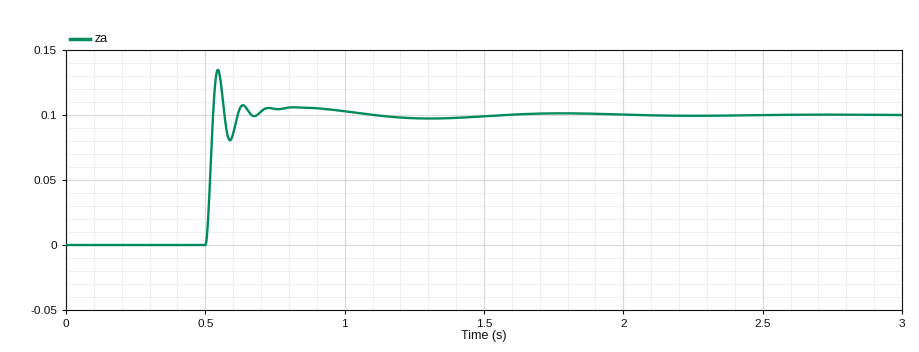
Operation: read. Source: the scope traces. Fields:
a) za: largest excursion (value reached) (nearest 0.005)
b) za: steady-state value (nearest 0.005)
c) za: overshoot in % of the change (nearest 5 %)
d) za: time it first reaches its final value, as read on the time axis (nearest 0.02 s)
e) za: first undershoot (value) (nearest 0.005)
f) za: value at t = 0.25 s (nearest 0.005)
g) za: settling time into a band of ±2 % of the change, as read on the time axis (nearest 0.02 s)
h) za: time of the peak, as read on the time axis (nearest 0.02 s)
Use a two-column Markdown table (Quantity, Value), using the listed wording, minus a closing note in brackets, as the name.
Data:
| Quantity | Value |
|---|---|
| za: largest excursion (value reached) | 0.135 |
| za: steady-state value | 0.100 |
| za: overshoot in % of the change | 35 % |
| za: time it first reaches its final value, as read on the time axis | 0.52 s |
| za: first undershoot (value) | 0.080 |
| za: value at t = 0.25 s | 0.000 |
| za: settling time into a band of ±2 % of the change, as read on the time axis | 1.42 s |
| za: time of the peak, as read on the time axis | 0.54 s |
